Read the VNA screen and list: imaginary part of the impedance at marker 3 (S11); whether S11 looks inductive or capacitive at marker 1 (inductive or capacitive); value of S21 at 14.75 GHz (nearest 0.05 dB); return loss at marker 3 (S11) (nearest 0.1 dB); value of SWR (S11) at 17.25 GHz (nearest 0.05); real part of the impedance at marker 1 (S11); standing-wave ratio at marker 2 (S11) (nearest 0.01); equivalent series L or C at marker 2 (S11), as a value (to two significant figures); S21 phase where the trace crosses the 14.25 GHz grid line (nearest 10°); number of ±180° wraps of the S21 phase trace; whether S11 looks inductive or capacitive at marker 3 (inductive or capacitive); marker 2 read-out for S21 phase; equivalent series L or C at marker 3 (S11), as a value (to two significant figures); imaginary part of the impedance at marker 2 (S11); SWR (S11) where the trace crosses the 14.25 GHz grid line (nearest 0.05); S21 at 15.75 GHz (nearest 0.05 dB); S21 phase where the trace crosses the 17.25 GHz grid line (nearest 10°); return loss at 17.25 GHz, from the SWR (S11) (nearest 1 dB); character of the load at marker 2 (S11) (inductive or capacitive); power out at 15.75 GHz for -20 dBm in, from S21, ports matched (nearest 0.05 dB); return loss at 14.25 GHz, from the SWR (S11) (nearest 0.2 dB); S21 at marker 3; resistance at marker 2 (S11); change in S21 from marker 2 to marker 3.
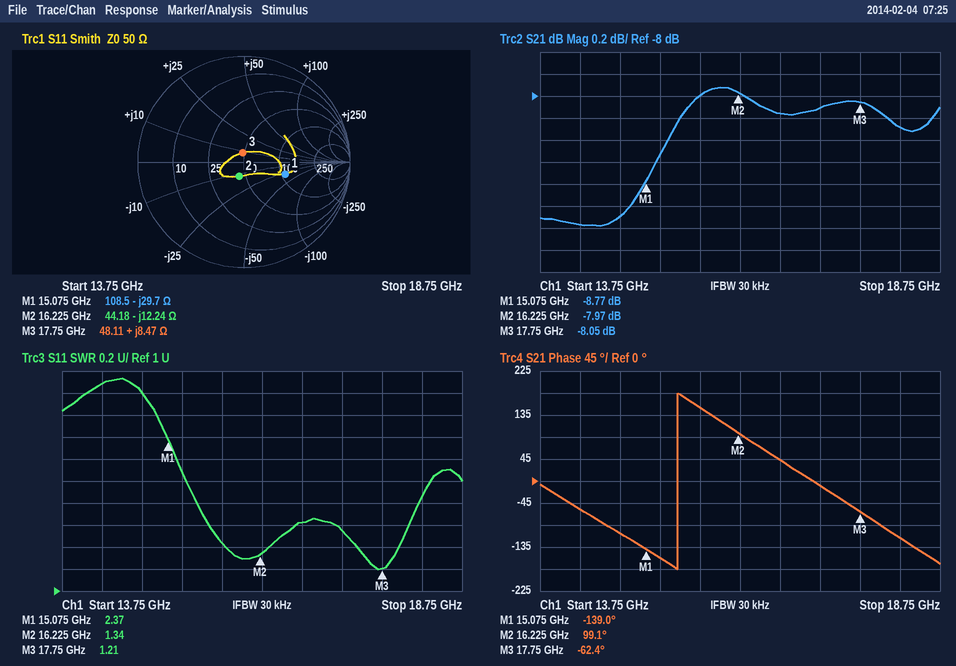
+8.47 Ω
capacitive
-9.10 dB
21.1 dB
1.55
108.5 Ω
1.33
800 fF
-60°
1
inductive
99.1°
76 pH
-12.24 Ω
2.90
-8.00 dB
-10°
13 dB
capacitive
-28.00 dBm
6.2 dB
-8.05 dB
44.18 Ω
-0.08 dB
